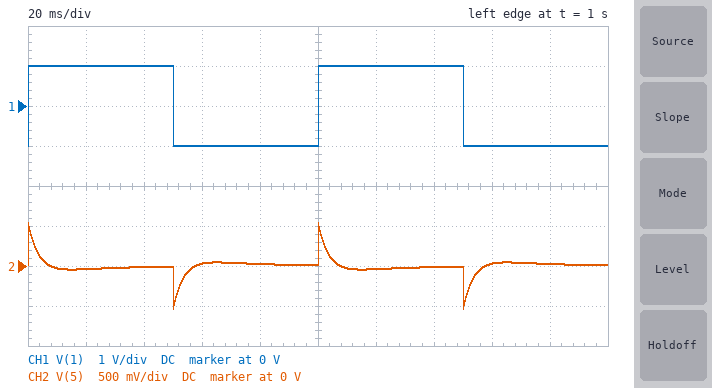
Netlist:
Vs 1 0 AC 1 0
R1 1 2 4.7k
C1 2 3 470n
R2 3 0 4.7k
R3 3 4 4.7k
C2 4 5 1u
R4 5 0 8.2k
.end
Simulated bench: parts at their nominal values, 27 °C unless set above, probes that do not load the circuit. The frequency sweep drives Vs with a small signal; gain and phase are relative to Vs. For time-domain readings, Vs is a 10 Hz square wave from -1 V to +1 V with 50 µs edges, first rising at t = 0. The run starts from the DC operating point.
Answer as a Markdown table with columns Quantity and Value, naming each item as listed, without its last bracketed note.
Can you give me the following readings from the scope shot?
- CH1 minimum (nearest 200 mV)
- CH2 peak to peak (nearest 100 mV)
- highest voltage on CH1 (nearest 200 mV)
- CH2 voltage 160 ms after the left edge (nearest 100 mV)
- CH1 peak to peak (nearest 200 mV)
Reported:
| Quantity | Value |
|---|---|
| CH1 minimum | -1.0 V |
| CH2 peak to peak | 1.1 V |
| highest voltage on CH1 | 1.0 V |
| CH2 voltage 160 ms after the left edge | 0 V |
| CH1 peak to peak | 2.0 V |
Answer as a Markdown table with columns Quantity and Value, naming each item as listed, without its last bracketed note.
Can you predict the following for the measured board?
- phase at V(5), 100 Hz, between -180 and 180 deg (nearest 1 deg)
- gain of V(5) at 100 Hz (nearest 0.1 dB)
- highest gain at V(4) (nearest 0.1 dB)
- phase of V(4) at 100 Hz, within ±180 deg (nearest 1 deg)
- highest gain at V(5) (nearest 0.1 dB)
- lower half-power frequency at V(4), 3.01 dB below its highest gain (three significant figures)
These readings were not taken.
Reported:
| Quantity | Value |
|---|---|
| phase at V(5), 100 Hz, between -180 and 180 deg | 28 deg |
| gain of V(5) at 100 Hz | -12.2 dB |
| highest gain at V(4) | -11.4 dB |
| phase of V(4) at 100 Hz, within ±180 deg | 17 deg |
| highest gain at V(5) | -11.4 dB |
| lower half-power frequency at V(4), 3.01 dB below its highest gain | 36.2 Hz |
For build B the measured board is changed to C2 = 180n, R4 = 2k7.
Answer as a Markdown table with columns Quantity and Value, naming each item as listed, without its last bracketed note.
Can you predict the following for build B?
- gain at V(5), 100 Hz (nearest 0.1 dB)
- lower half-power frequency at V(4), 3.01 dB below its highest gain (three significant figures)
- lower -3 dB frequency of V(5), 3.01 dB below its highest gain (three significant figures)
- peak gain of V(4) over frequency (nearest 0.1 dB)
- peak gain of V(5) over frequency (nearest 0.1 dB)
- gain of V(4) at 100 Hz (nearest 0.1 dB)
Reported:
| Quantity | Value |
|---|---|
| gain at V(5), 100 Hz | -20.8 dB |
| lower half-power frequency at V(4), 3.01 dB below its highest gain | 21.3 Hz |
| lower -3 dB frequency of V(5), 3.01 dB below its highest gain | 112 Hz |
| peak gain of V(4) over frequency | -9.4 dB |
| peak gain of V(5) over frequency | -17.2 dB |
| gain of V(4) at 100 Hz | -10.1 dB |
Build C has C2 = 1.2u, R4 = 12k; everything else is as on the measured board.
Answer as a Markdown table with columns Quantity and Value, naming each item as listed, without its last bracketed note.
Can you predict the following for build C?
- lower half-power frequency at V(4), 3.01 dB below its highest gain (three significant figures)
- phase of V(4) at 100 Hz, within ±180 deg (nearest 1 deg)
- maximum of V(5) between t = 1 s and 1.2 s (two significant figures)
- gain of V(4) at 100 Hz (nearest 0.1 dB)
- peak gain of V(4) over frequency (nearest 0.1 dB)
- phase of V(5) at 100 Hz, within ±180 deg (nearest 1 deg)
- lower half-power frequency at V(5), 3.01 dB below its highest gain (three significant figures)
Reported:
| Quantity | Value |
|---|---|
| lower half-power frequency at V(4), 3.01 dB below its highest gain | 39.3 Hz |
| phase of V(4) at 100 Hz, within ±180 deg | 20 deg |
| maximum of V(5) between t = 1 s and 1.2 s | 640 mV |
| gain of V(4) at 100 Hz | -10.7 dB |
| peak gain of V(4) over frequency | -10.0 dB |
| phase of V(5) at 100 Hz, within ±180 deg | 26 deg |
| lower half-power frequency at V(5), 3.01 dB below its highest gain | 42.2 Hz |
